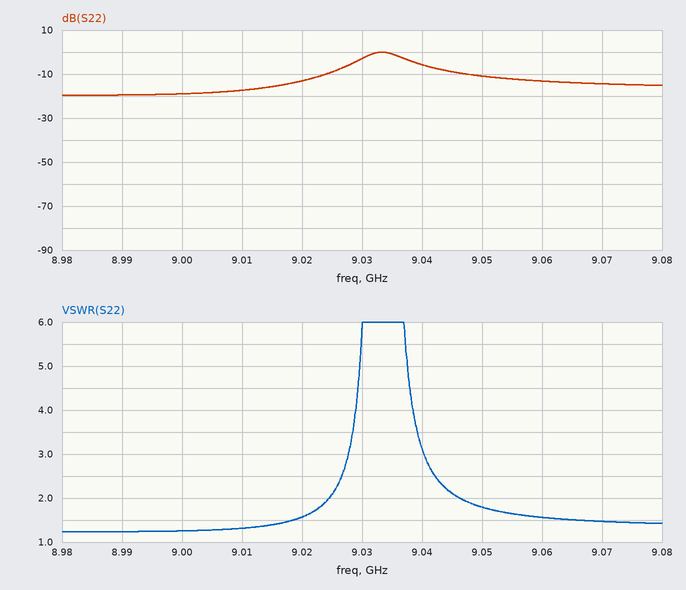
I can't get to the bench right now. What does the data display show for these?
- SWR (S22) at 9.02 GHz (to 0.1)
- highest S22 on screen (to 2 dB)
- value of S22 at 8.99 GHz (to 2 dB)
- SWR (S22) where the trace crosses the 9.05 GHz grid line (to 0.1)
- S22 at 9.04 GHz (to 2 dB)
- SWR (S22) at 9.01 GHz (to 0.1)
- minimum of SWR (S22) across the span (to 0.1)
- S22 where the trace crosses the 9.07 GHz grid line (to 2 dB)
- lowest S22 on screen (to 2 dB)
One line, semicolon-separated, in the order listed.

1.6; 0 dB; -20 dB; 1.8; -6 dB; 1.3; 1.2; -14 dB; -20 dB
